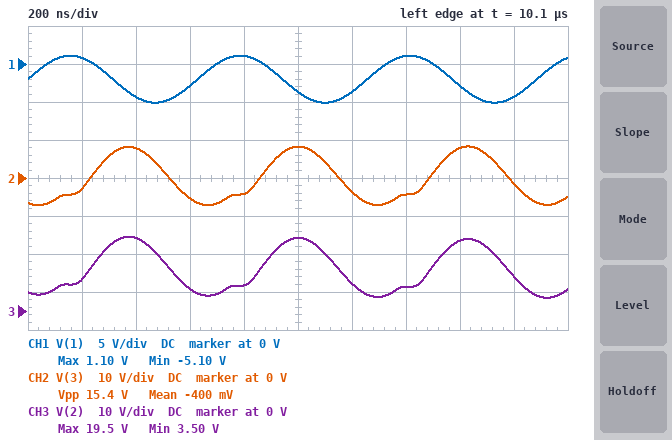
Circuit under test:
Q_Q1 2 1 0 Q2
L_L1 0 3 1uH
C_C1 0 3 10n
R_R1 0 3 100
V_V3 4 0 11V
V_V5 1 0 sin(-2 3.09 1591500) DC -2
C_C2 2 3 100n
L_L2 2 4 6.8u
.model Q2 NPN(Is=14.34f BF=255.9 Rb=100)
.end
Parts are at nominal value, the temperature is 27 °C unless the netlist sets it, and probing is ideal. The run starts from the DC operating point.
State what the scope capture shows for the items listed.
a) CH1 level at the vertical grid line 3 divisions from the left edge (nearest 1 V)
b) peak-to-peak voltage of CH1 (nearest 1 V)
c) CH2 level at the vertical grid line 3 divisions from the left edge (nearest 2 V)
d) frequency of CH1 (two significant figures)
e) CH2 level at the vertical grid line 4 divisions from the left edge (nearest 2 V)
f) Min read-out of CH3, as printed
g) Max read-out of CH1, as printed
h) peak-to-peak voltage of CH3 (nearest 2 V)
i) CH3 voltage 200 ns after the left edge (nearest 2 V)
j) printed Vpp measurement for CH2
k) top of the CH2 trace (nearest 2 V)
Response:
-3 V
6 V
-6 V
1.6 MHz
-4 V
3.50 V
1.10 V
16 V
8 V
15.4 V
8 V
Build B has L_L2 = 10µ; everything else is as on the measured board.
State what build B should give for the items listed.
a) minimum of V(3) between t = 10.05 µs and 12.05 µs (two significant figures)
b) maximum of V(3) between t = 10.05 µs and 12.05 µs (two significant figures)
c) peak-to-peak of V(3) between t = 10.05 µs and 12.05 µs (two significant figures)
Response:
-8.8 V
10 V
19 V
